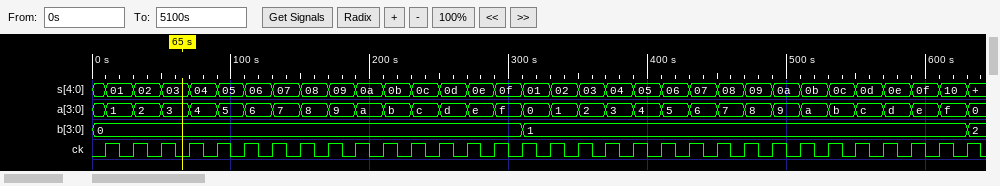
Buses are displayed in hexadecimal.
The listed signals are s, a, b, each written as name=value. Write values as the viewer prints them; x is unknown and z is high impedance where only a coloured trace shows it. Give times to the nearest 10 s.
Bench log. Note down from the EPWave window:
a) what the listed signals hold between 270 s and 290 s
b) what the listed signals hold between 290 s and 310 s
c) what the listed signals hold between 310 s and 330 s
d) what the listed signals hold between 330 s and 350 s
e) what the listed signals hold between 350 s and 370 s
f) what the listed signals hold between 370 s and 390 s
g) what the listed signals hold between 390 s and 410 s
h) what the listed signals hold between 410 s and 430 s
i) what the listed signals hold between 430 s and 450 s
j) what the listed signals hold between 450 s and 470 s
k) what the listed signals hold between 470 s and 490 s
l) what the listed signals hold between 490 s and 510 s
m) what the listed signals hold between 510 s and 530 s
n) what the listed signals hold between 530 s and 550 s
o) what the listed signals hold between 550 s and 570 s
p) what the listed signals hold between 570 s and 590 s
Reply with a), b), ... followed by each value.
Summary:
a) s=0e, a=e, b=0
b) s=0f, a=f, b=0
c) s=01, a=0, b=1
d) s=02, a=1, b=1
e) s=03, a=2, b=1
f) s=04, a=3, b=1
g) s=05, a=4, b=1
h) s=06, a=5, b=1
i) s=07, a=6, b=1
j) s=08, a=7, b=1
k) s=09, a=8, b=1
l) s=0a, a=9, b=1
m) s=0b, a=a, b=1
n) s=0c, a=b, b=1
o) s=0d, a=c, b=1
p) s=0e, a=d, b=1
